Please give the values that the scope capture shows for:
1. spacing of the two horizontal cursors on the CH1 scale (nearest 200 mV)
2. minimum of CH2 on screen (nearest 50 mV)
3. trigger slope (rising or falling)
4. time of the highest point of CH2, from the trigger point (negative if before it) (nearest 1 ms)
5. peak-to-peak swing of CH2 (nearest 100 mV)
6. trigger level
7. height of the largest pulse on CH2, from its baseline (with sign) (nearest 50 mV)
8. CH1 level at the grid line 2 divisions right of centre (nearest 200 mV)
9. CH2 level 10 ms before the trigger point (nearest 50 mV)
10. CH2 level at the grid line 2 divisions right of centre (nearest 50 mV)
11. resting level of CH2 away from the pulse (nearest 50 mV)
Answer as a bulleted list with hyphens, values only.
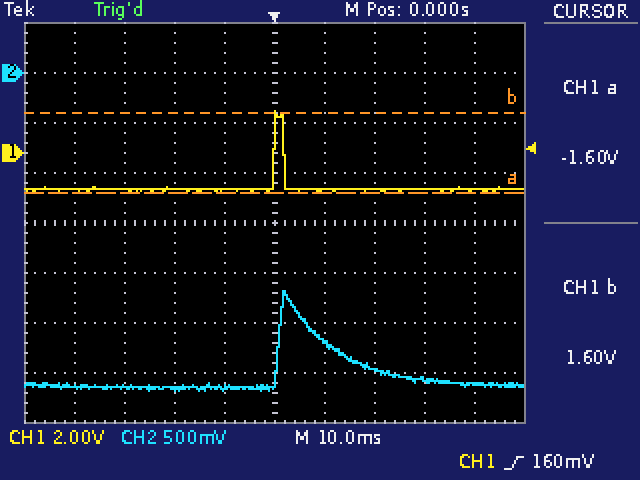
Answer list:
- 3.2 V
- -3.20 V
- rising
- +2 ms
- 1.00 V
- 160 mV
- +950 mV
- -1.4 V
- -3.15 V
- -2.95 V
- -3.15 V
